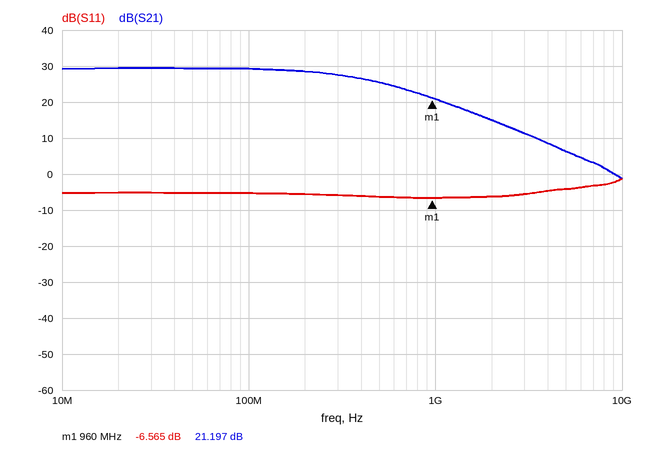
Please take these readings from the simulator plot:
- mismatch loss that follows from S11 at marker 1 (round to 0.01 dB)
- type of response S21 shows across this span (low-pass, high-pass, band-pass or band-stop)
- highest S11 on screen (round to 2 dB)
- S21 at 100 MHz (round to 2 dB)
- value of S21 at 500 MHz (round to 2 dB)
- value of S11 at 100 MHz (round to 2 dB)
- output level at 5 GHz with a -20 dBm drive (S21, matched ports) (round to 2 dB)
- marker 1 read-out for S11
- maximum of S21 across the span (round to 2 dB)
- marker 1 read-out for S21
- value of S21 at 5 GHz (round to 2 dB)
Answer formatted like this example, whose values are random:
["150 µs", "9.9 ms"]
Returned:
["1.08 dB", "low-pass", "-2 dB", "30 dB", "26 dB", "-6 dB", "-14 dBm", "-6.565 dB", "30 dB", "21.197 dB", "6 dB"]
